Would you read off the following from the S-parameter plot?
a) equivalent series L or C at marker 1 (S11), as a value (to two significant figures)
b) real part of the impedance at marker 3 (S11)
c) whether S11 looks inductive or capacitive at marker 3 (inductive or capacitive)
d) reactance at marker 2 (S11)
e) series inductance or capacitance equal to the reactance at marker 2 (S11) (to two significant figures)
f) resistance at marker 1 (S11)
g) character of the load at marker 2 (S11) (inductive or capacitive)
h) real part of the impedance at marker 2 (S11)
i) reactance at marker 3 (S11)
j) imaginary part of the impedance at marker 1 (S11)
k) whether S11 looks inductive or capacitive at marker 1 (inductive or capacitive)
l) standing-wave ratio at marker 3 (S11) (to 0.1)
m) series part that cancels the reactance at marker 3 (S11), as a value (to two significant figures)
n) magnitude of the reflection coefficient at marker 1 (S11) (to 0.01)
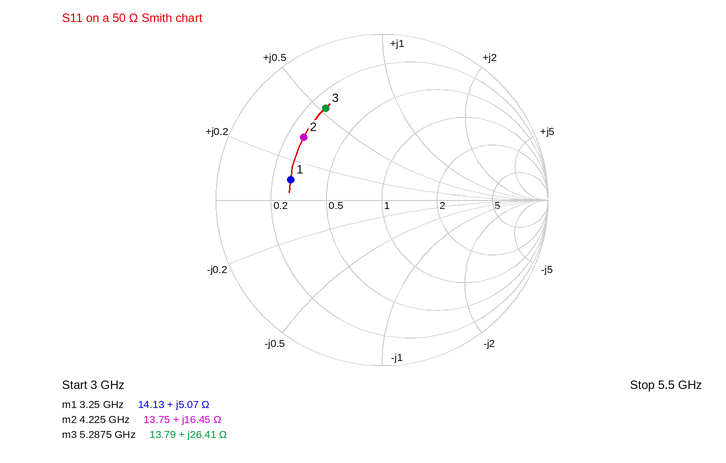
250 pH
13.79 Ω
inductive
+16.45 Ω
620 pH
14.13 Ω
inductive
13.75 Ω
+26.41 Ω
+5.07 Ω
inductive
4.7
1.1 pF
0.56
